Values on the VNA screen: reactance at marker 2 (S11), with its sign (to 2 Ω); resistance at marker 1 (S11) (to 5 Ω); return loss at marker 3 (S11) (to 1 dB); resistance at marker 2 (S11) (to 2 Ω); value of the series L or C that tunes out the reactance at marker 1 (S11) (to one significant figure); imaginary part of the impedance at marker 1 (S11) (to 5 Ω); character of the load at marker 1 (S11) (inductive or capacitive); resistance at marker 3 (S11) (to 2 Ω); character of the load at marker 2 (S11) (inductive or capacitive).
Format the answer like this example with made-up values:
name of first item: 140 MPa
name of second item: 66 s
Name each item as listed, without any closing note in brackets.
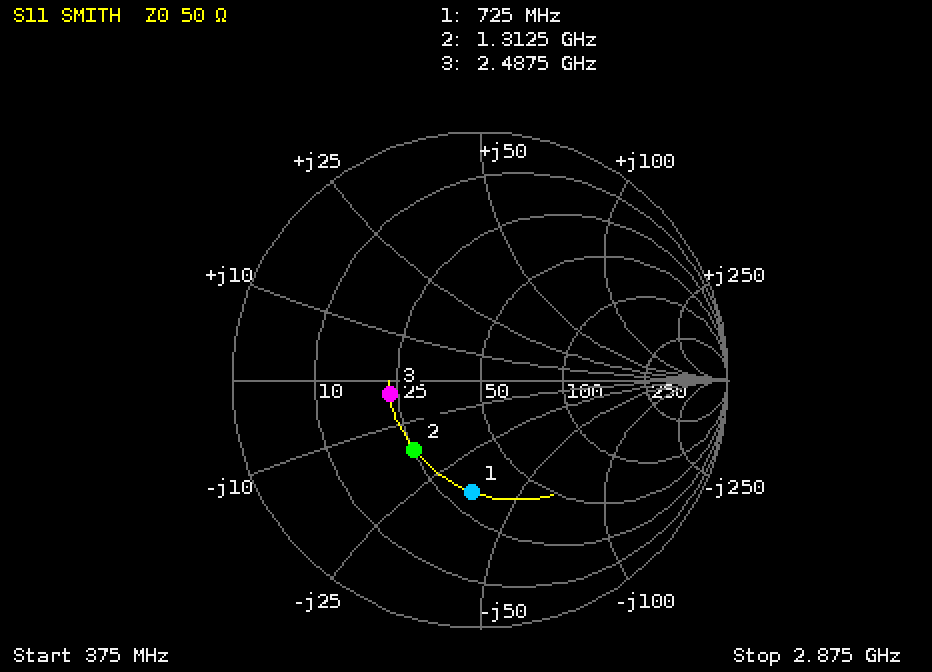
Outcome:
reactance at marker 2 (S11), with its sign: -16 Ω
resistance at marker 1 (S11): 30 Ω
return loss at marker 3 (S11): 9 dB
resistance at marker 2 (S11): 26 Ω
value of the series L or C that tunes out the reactance at marker 1 (S11): 8 nH
imaginary part of the impedance at marker 1 (S11): -35 Ω
character of the load at marker 1 (S11): capacitive
resistance at marker 3 (S11): 24 Ω
character of the load at marker 2 (S11): capacitive
